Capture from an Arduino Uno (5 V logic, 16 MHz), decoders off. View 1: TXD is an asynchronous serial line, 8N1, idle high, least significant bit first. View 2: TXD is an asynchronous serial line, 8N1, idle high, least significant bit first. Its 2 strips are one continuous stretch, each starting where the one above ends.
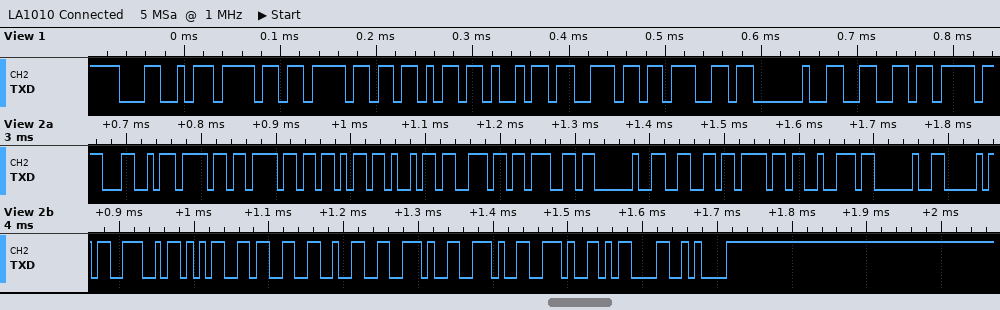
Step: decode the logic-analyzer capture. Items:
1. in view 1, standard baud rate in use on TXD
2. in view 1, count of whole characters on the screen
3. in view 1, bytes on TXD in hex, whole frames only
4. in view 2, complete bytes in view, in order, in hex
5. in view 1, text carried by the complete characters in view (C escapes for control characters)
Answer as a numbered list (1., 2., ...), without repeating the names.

1. 115200 baud
2. 9
3. 4C 6F 6F 6B 69 6E 67 20 66
4. 0x4C 0x6F 0x6F 0x6B 0x69 0x6E 0x67 0x20 0x66 0x6F 0x72 0x20 0x50 0x4E 0x35 0x33 0x32 0x2E 0x2E 0x2E 0x0D 0x0A
5. "Looking f"
